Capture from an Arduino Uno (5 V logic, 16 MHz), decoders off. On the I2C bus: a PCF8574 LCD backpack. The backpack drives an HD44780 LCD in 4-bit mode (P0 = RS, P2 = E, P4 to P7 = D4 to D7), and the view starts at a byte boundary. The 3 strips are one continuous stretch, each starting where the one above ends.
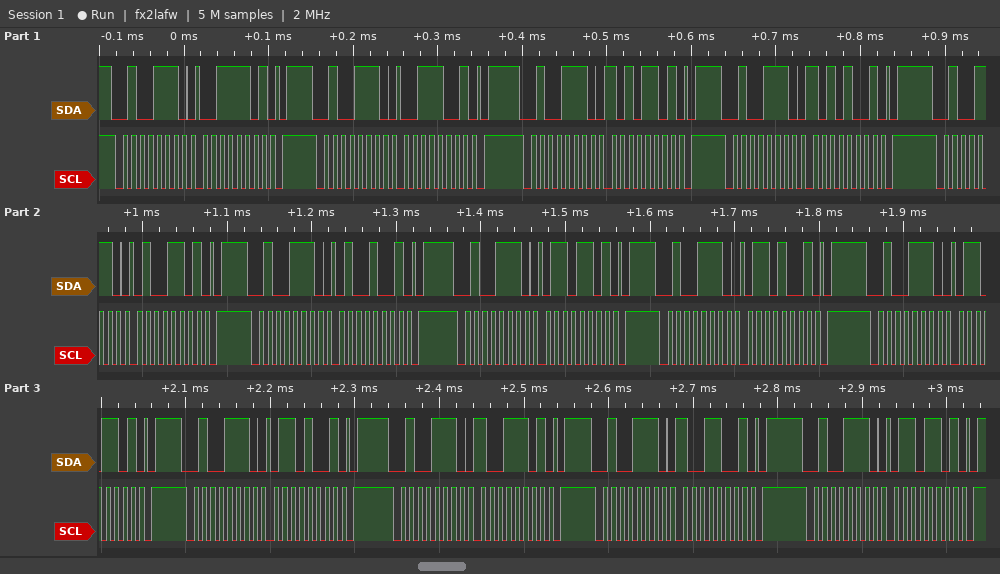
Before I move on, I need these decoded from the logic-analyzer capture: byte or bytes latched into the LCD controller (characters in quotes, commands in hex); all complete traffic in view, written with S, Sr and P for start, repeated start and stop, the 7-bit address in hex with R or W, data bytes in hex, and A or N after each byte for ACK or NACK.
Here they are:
':' 'F' 'i'
S 27W A 3D A P S 27W A 39 A P S 27W A AD A P S 27W A A9 A P S 27W A 4D A P S 27W A 49 A P S 27W A 6D A P S 27W A 69 A P S 27W A 6D A P S 27W A 69 A P S 27W A 9D A P S 27W A 99 A P S 27W A 6D A P
